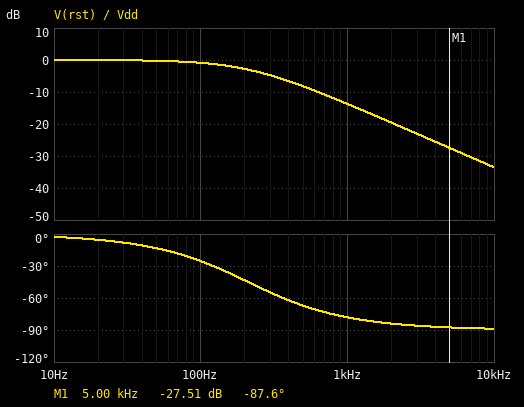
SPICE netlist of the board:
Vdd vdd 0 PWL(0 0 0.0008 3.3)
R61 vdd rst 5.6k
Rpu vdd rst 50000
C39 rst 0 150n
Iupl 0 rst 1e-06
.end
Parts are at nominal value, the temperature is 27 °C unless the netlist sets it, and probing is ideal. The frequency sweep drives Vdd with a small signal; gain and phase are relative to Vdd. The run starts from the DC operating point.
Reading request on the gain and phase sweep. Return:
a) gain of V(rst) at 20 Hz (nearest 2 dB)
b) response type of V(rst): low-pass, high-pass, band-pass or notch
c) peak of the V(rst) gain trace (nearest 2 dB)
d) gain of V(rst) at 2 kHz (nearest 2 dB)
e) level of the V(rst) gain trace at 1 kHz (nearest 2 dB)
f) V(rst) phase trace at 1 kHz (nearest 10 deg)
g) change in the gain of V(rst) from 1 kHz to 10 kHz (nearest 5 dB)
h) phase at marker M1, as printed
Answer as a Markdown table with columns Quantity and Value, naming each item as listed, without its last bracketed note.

| Quantity | Value |
|---|---|
| gain of V(rst) at 20 Hz | 0 dB |
| response type of V(rst): low-pass, high-pass, band-pass or notch | low-pass |
| peak of the V(rst) gain trace | 0 dB |
| gain of V(rst) at 2 kHz | -20 dB |
| level of the V(rst) gain trace at 1 kHz | -14 dB |
| V(rst) phase trace at 1 kHz | -80 deg |
| change in the gain of V(rst) from 1 kHz to 10 kHz | -20 dB |
| phase at marker M1, as printed | -87.6 deg |
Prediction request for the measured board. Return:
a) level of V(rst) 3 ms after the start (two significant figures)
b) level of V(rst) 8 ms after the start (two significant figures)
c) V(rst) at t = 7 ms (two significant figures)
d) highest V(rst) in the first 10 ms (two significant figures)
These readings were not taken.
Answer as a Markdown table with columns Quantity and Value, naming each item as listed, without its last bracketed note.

| Quantity | Value |
|---|---|
| level of V(rst) 3 ms after the start | 3.2 V |
| level of V(rst) 8 ms after the start | 3.3 V |
| V(rst) at t = 7 ms | 3.3 V |
| highest V(rst) in the first 10 ms | 3.3 V |
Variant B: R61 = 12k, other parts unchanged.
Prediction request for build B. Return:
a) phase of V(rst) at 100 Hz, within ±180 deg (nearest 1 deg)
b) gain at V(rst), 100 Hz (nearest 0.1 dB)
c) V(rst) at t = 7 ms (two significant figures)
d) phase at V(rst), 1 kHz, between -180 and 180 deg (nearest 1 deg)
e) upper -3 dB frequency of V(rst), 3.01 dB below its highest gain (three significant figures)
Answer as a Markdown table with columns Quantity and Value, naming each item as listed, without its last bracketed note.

| Quantity | Value |
|---|---|
| phase of V(rst) at 100 Hz, within ±180 deg | -42 deg |
| gain at V(rst), 100 Hz | -2.6 dB |
| V(rst) at t = 7 ms | 3.3 V |
| phase at V(rst), 1 kHz, between -180 and 180 deg | -84 deg |
| upper -3 dB frequency of V(rst), 3.01 dB below its highest gain | 110 Hz |
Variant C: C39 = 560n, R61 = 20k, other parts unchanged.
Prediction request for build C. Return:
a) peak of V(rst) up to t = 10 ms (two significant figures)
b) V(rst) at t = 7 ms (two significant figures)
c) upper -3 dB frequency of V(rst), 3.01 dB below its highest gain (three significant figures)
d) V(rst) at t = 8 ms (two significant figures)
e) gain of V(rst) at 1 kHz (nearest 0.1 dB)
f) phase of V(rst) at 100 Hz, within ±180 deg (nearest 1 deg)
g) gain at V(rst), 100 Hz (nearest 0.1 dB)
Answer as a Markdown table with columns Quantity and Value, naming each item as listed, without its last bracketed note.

| Quantity | Value |
|---|---|
| peak of V(rst) up to t = 10 ms | 2.3 V |
| V(rst) at t = 7 ms | 1.9 V |
| upper -3 dB frequency of V(rst), 3.01 dB below its highest gain | 19.9 Hz |
| V(rst) at t = 8 ms | 2.0 V |
| gain of V(rst) at 1 kHz | -34.0 dB |
| phase of V(rst) at 100 Hz, within ±180 deg | -79 deg |
| gain at V(rst), 100 Hz | -14.2 dB |
